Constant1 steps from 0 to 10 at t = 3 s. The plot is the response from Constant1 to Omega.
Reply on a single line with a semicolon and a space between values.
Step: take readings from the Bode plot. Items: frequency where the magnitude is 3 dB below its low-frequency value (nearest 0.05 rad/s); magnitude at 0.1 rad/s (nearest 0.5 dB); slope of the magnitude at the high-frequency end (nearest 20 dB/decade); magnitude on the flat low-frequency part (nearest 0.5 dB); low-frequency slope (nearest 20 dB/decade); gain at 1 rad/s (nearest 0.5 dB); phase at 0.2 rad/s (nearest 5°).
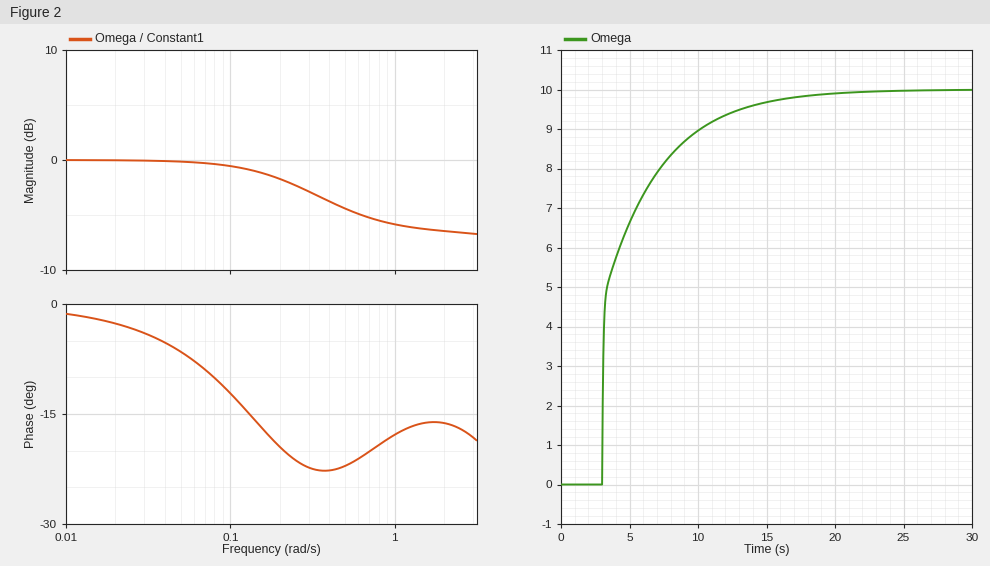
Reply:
0.30 rad/s; -0.5 dB; 0 dB/decade; 0.0 dB; 0 dB/decade; -6.0 dB; -20°
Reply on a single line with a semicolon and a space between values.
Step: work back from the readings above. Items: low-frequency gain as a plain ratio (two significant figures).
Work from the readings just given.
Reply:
1.0
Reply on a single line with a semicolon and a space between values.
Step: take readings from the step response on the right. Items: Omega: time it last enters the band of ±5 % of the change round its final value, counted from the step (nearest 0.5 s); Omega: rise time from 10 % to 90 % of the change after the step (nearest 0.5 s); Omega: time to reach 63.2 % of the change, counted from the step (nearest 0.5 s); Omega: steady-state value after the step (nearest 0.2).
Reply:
10.0 s; 7.0 s; 1.5 s; 10.0
